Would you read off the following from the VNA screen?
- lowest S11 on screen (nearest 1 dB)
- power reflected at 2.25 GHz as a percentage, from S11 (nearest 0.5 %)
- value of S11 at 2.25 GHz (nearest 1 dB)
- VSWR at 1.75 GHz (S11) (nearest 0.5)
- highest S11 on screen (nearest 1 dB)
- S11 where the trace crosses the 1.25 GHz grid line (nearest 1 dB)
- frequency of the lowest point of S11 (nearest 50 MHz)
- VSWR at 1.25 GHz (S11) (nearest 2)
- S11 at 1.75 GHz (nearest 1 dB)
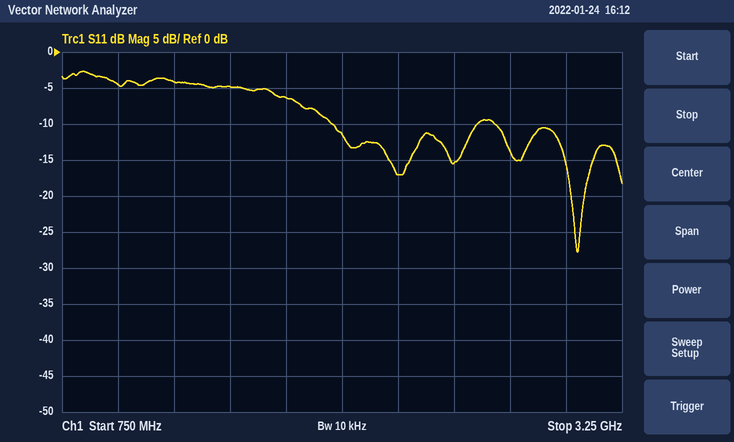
-28 dB
2.0 %
-17 dB
3.0
-3 dB
-4 dB
3.05 GHz
4
-6 dB
